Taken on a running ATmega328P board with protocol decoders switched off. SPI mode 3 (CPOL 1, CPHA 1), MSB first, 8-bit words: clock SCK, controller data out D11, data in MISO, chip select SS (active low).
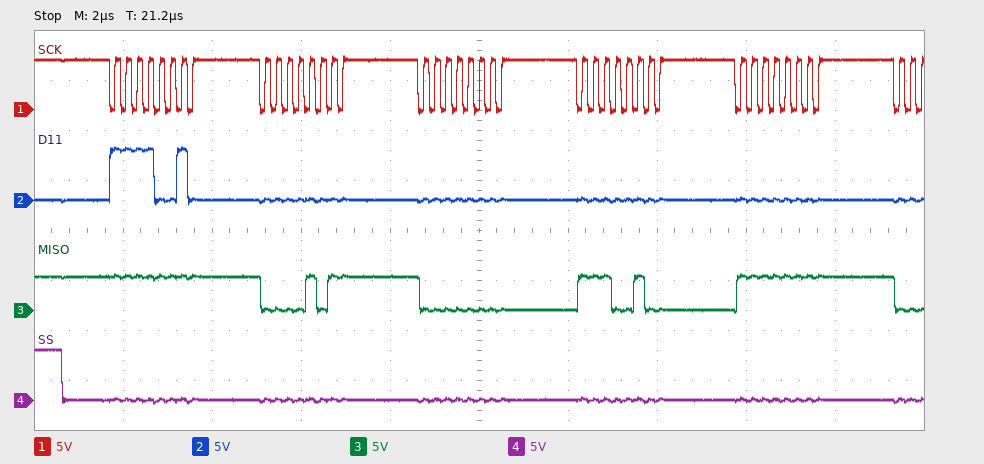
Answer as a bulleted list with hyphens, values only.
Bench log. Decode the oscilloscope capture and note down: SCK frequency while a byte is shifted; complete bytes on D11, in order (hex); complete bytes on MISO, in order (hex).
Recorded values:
- 4 MHz
- F2 00 00 00 00
- FF 0B 00 E4 FF
